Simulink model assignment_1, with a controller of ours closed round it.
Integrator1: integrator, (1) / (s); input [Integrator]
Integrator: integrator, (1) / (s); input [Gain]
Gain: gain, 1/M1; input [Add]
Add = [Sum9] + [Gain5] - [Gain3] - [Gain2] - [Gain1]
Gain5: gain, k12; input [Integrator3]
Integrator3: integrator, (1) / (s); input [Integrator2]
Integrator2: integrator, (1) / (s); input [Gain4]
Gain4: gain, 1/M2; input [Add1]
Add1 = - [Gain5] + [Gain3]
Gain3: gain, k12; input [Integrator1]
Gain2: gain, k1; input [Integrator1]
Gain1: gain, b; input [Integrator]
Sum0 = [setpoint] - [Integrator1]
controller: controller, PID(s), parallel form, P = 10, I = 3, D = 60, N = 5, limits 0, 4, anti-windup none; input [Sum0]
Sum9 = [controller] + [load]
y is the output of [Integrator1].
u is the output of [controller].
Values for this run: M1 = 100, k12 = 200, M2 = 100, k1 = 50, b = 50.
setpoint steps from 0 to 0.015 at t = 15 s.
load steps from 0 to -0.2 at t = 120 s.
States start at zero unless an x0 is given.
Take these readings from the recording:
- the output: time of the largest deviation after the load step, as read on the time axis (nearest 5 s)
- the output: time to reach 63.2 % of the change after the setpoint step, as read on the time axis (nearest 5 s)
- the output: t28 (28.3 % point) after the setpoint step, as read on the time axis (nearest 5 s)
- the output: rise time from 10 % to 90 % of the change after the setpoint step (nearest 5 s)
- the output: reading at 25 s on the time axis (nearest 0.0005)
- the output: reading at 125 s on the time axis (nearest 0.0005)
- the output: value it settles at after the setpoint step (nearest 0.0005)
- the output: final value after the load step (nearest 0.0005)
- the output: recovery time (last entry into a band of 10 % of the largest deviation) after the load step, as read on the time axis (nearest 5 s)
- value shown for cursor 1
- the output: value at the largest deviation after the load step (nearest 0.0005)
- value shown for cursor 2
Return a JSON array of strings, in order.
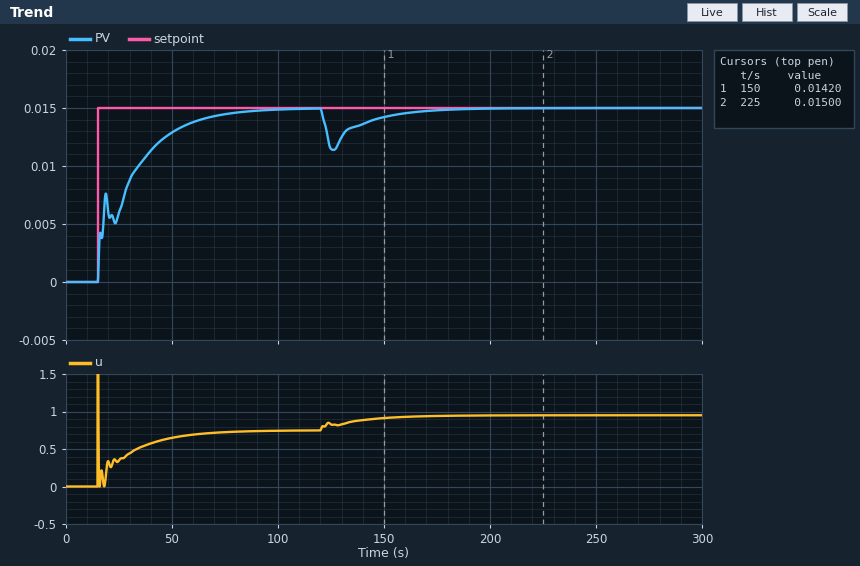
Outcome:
["125 s", "30 s", "15 s", "40 s", "0.0060", "0.0115", "0.0150", "0.0150", "165 s", "0.01420", "0.0115", "0.01500"]
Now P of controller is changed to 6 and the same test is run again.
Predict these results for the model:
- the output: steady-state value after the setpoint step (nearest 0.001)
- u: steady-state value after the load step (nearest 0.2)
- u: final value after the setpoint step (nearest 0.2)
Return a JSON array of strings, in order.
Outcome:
["0.015", "1.0", "0.8"]
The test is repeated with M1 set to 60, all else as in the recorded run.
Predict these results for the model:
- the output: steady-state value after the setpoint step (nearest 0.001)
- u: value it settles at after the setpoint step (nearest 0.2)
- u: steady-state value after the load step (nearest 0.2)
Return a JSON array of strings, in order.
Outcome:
["0.015", "0.8", "1.0"]
